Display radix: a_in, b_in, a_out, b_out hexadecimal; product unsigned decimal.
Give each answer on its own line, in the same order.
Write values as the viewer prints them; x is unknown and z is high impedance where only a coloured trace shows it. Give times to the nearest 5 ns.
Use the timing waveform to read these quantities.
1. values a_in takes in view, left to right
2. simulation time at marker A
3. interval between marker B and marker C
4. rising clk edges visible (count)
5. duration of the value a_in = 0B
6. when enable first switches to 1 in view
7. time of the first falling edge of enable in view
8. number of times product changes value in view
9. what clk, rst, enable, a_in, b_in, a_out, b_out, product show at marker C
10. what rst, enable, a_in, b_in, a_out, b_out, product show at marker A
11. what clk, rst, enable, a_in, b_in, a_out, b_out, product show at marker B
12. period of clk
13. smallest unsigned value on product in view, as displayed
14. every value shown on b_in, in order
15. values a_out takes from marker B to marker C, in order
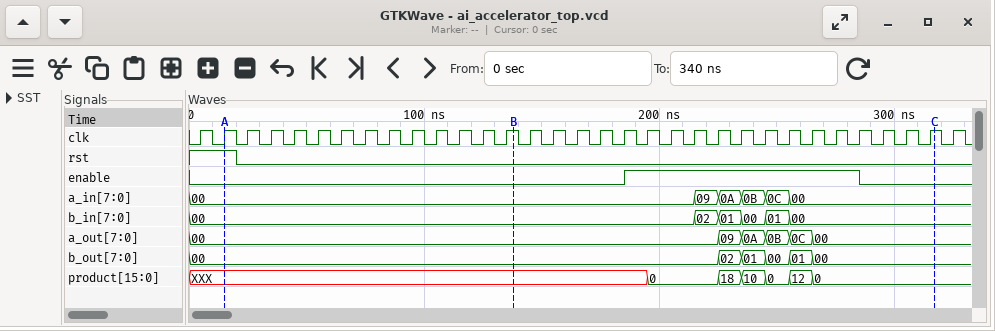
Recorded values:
00, 09, 0A, 0B, 0C, 00
15 ns
180 ns
33
10 ns
185 ns
285 ns
6
clk=1, rst=0, enable=0, a_in=00, b_in=00, a_out=00, b_out=00, product=0
rst=1, enable=0, a_in=00, b_in=00, a_out=00, b_out=00, product=XXX
clk=1, rst=0, enable=0, a_in=00, b_in=00, a_out=00, b_out=00, product=XXX
10 ns
0
00, 02, 01, 00, 01, 00
00, 09, 0A, 0B, 0C, 00
